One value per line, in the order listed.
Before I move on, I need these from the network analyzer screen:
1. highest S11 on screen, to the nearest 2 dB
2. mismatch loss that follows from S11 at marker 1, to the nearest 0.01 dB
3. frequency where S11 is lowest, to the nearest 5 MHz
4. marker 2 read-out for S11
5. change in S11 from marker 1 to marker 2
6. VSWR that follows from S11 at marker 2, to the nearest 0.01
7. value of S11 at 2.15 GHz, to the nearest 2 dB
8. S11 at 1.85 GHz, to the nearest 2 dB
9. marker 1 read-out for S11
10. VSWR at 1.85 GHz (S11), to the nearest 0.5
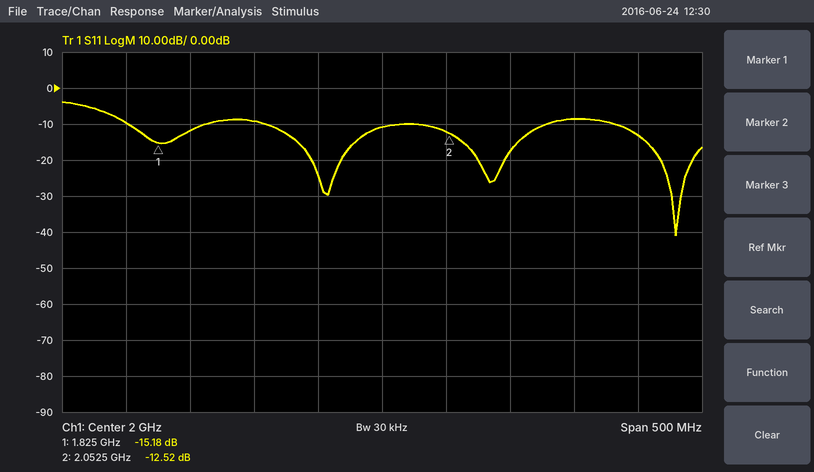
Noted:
-4 dB
0.13 dB
2.230 GHz
-12.52 dB
2.66 dB
1.62
-8 dB
-12 dB
-15.18 dB
1.5
